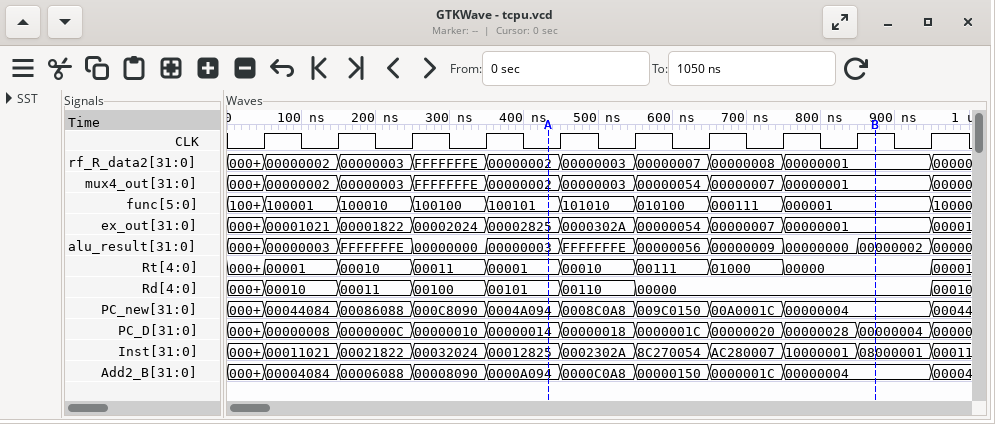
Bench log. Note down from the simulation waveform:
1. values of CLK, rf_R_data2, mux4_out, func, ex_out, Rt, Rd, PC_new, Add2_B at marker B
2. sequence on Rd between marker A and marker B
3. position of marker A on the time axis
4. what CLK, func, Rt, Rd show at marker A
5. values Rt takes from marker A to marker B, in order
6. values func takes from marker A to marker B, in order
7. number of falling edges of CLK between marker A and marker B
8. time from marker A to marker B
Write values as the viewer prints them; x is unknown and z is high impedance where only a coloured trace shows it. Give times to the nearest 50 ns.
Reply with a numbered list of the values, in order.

1. CLK=1, rf_R_data2=00000001, mux4_out=00000001, func=000001, ex_out=00000001, Rt=00000, Rd=00000, PC_new=00000004, Add2_B=00000004
2. 00101, 00110, 00000
3. 450 ns
4. CLK=0, func=100101, Rt=00001, Rd=00101
5. 00001, 00010, 00111, 01000, 00000
6. 100101, 101010, 010100, 000111, 000001
7. 4
8. 450 ns
